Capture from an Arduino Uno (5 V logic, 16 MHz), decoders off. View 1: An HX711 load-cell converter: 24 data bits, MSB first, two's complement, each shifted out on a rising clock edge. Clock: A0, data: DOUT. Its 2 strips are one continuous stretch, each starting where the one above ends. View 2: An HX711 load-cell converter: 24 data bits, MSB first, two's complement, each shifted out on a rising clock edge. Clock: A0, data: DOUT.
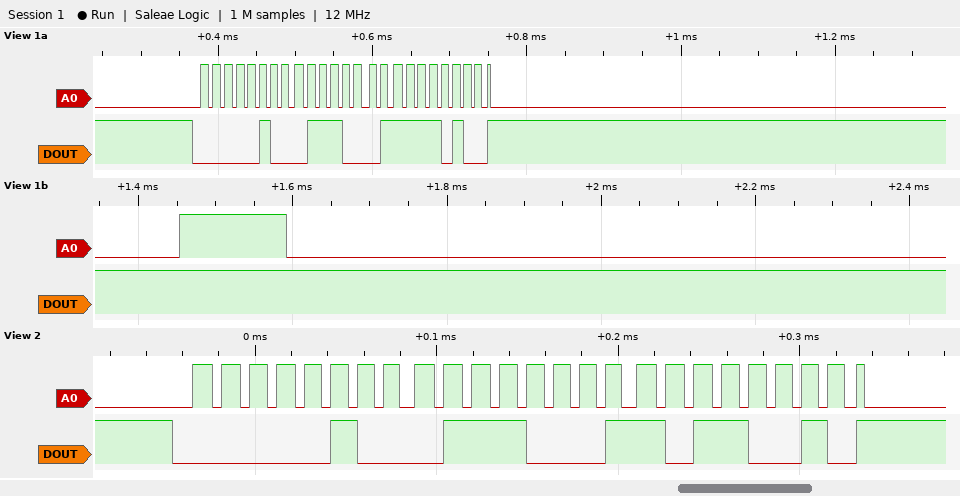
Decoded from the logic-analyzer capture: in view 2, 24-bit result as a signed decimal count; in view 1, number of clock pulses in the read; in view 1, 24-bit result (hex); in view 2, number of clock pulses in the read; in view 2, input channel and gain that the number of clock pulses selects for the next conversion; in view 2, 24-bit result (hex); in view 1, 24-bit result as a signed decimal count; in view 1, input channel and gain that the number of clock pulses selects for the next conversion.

291250
26
0x0471F4
25
channel A, gain 128
0x0471B2
291316
channel B, gain 32
